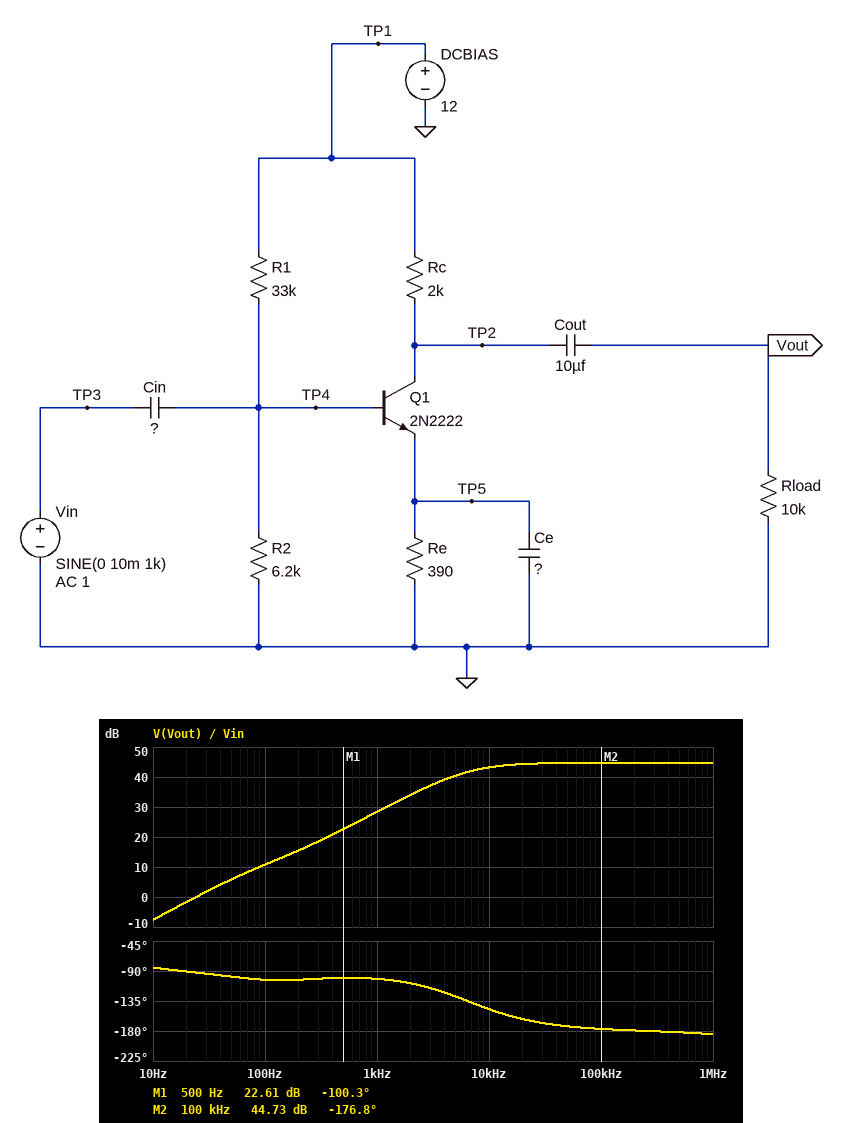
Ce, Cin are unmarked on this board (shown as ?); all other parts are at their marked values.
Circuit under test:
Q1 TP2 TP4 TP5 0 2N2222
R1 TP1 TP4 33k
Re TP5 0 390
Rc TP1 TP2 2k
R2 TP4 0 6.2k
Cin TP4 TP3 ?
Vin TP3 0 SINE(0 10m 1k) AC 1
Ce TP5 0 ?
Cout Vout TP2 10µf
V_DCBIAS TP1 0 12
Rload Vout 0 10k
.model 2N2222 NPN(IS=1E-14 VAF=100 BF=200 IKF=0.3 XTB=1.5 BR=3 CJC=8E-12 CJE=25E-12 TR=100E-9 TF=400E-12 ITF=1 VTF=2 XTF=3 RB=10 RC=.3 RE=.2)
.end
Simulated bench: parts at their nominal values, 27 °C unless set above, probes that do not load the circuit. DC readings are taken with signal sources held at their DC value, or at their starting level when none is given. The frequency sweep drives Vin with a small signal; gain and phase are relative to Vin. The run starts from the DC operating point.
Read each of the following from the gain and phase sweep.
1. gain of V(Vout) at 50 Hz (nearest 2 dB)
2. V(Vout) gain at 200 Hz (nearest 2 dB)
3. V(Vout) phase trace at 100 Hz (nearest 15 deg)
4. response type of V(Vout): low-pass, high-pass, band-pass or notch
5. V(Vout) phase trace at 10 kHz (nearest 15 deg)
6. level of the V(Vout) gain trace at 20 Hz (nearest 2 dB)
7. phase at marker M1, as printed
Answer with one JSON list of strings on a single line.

["6 dB", "16 dB", "-105 deg", "high-pass", "-150 deg", "-2 dB", "-100.3 deg"]
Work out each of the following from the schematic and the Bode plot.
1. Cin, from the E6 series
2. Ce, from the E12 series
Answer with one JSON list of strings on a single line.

["330 nF", "2.7 µF"]
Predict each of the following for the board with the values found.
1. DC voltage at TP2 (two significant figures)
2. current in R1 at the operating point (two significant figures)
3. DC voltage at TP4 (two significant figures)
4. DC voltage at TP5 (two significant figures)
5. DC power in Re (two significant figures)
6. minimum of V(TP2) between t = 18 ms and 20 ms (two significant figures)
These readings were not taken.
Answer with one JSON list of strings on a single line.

["6.2 V", "310 µA", "1.8 V", "1.1 V", "3.3 mW", "5.9 V"]
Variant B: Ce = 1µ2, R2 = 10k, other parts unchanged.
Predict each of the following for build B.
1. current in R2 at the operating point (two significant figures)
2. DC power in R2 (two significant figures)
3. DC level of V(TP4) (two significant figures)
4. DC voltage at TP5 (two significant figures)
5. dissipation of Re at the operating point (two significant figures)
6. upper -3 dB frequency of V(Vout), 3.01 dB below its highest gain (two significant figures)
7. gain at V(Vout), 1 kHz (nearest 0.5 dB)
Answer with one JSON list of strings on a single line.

["260 µA", "680 µW", "2.6 V", "1.9 V", "9.3 mW", "3.9 MHz", "22.0 dB"]
